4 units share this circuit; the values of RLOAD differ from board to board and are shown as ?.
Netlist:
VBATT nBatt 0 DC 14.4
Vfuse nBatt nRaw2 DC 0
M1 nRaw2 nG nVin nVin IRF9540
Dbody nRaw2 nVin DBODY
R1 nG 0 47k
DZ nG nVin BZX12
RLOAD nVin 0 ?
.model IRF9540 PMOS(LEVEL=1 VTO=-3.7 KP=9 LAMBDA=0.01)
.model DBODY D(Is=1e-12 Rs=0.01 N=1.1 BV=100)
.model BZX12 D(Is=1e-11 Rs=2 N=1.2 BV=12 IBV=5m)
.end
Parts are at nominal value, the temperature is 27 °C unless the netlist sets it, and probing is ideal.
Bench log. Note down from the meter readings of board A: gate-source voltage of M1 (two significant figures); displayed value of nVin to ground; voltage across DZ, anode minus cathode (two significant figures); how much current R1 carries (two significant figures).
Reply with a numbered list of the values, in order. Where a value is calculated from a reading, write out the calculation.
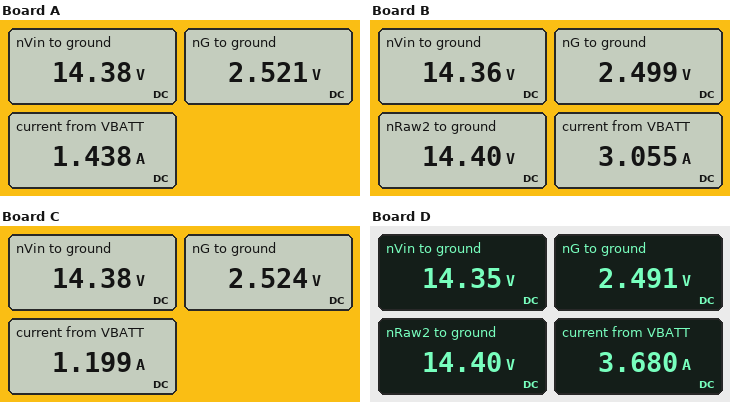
1. 2.521 V - 14.38 V = -12 V
2. 14.38 V
3. 2.521 V - 14.38 V = -12 V
4. (2.521 V) / 47 kΩ = 54 µA
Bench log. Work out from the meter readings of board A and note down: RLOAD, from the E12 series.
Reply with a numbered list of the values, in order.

1. 10 Ω
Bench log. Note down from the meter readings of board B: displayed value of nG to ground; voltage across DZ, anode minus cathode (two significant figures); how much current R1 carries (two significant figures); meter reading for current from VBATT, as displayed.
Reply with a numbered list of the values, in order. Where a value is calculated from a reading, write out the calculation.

1. 2.499 V
2. 2.499 V - 14.36 V = -12 V
3. (2.499 V) / 47 kΩ = 53 µA
4. 3.055 A
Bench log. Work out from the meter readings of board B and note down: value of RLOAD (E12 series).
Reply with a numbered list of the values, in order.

1. 4.7 Ω
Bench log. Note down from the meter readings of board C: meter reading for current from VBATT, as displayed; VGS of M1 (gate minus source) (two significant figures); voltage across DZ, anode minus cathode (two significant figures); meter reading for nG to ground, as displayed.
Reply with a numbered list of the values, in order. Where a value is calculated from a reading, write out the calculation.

1. 1.199 A
2. 2.524 V - 14.38 V = -12 V
3. 2.524 V - 14.38 V = -12 V
4. 2.524 V
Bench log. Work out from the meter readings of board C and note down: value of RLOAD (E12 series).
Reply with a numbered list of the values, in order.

1. 12 Ω
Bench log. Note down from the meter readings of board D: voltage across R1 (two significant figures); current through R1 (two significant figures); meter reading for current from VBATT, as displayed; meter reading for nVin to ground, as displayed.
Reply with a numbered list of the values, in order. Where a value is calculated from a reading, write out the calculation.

1. 2.491 V = 2.5 V
2. (2.491 V) / 47 kΩ = 53 µA
3. 3.680 A
4. 14.35 V
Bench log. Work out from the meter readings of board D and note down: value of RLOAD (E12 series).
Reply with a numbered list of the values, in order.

1. 3.9 Ω
